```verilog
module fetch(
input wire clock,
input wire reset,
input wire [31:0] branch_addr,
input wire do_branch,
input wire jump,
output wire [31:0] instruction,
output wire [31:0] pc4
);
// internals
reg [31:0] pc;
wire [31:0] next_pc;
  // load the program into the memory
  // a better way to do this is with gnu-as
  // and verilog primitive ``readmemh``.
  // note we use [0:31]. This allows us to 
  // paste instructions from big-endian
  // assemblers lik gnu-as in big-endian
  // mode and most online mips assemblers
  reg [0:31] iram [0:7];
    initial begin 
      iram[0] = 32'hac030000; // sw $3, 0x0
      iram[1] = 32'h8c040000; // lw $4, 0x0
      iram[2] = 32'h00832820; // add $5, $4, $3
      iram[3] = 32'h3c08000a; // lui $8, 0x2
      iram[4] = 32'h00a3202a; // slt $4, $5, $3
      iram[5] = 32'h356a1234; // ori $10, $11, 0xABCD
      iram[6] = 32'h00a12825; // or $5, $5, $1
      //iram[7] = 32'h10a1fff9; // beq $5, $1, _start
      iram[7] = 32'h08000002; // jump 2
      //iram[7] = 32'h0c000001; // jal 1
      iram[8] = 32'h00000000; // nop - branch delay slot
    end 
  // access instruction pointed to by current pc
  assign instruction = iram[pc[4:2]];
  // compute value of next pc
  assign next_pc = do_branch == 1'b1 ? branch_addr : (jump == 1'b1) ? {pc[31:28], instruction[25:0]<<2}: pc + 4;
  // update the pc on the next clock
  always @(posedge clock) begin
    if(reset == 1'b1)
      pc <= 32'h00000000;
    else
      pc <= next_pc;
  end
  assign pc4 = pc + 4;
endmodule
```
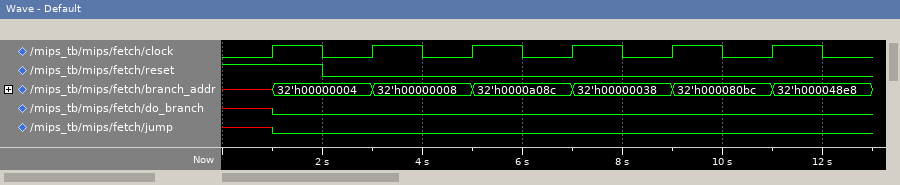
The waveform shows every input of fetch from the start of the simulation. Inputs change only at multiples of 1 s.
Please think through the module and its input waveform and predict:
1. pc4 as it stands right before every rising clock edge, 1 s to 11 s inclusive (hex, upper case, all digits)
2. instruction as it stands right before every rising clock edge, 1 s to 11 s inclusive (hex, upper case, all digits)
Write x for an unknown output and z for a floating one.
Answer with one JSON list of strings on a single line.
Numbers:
["x, 00000004, 00000008, 0000000C, 00000010, 00000014", "x, AC030000, 8C040000, 00832820, 3C08000A, 00A3202A"]
